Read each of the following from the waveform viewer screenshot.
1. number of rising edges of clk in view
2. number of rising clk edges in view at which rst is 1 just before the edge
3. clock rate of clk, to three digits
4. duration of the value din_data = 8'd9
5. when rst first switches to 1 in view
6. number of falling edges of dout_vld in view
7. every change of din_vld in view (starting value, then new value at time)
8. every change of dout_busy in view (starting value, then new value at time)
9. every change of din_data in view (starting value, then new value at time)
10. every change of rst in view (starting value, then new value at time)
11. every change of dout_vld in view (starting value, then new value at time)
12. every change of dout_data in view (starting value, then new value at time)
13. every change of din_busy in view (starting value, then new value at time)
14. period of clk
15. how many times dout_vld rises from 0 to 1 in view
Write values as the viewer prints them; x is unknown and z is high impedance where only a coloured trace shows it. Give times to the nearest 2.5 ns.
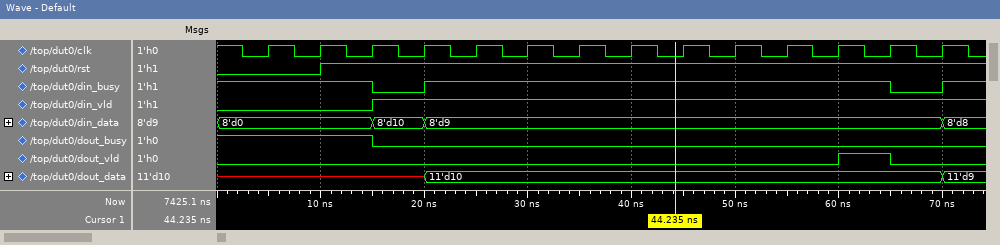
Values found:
14
12
200 MHz
50 ns
10 ns
1
0, 1 at 15 ns
1, 0 at 15 ns
8'd0, 8'd10 at 15 ns, 8'd9 at 20 ns, 8'd8 at 70 ns
0, 1 at 10 ns
0, 1 at 60 ns, 0 at 65 ns
x, 11'd10 at 20 ns, 11'd9 at 70 ns
1, 0 at 15 ns, 1 at 20 ns, 0 at 65 ns, 1 at 70 ns
5 ns
1
